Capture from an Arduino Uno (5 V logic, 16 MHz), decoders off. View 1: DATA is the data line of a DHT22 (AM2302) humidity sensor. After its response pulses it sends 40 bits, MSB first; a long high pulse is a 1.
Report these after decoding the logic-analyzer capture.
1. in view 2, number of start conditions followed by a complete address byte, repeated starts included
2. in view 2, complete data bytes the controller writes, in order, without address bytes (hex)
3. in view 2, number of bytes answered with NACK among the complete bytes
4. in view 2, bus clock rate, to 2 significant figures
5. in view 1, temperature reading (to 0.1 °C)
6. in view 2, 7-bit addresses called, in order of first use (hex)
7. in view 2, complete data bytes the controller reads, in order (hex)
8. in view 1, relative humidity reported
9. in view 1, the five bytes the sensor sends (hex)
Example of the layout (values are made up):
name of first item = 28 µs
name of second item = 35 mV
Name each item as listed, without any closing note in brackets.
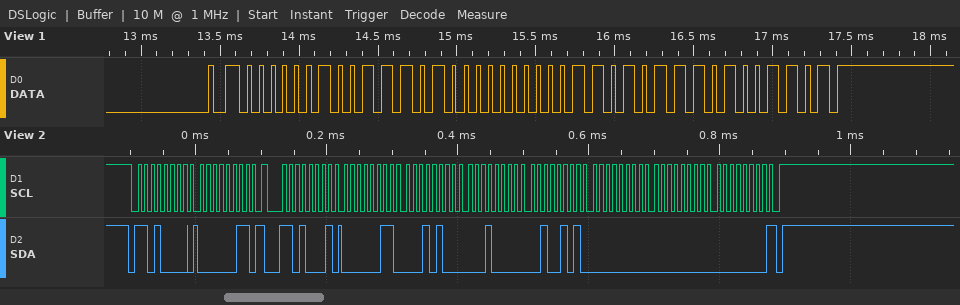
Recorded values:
in view 2, number of start conditions followed by a complete address byte, repeated starts included = 2
in view 2, complete data bytes the controller writes, in order, without address bytes = 03
in view 2, number of bytes answered with NACK among the complete bytes = 1
in view 2, bus clock rate, to 2 significant figures = 100 kHz
in view 1, temperature reading = 21.5 °C
in view 2, 7-bit addresses called, in order of first use = 0x68
in view 2, complete data bytes the controller reads, in order = 03 14 10 25 00 00 00
in view 1, relative humidity reported = 62.8 %
in view 1, the five bytes the sensor sends = 02 74 00 D7 4D
